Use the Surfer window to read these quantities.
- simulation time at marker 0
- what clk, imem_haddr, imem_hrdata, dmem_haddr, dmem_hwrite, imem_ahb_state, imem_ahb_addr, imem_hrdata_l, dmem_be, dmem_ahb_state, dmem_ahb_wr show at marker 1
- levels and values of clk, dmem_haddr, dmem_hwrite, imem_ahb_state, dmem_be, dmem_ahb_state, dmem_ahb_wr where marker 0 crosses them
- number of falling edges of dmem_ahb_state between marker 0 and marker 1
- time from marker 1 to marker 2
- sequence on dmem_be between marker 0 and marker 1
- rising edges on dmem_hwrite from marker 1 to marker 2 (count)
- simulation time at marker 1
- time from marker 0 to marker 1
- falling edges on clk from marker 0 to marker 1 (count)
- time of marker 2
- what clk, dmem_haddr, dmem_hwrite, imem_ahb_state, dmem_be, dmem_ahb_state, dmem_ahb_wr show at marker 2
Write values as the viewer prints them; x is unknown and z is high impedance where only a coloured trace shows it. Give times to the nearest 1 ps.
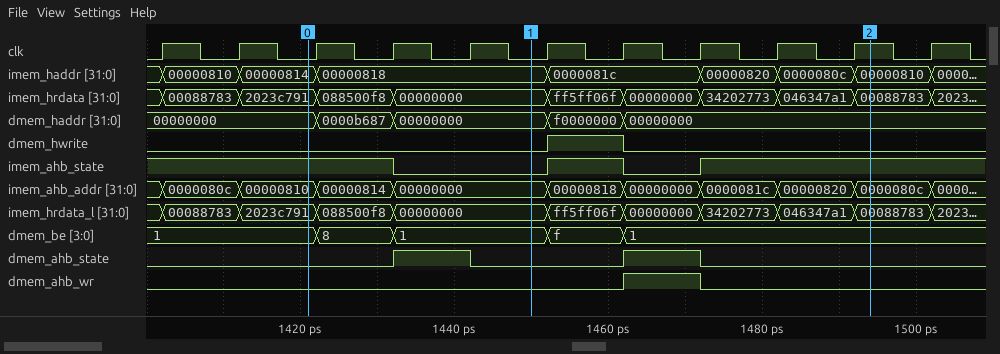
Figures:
1421 ps
clk=0, imem_haddr=00000818, imem_hrdata=00000000, dmem_haddr=00000000, dmem_hwrite=0, imem_ahb_state=0, imem_ahb_addr=00000000, imem_hrdata_l=00000000, dmem_be=1, dmem_ahb_state=0, dmem_ahb_wr=0
clk=0, dmem_haddr=00000000, dmem_hwrite=0, imem_ahb_state=1, dmem_be=1, dmem_ahb_state=0, dmem_ahb_wr=0
1
44 ps
1, 8, 1
1
1450 ps
29 ps
3
1494 ps
clk=1, dmem_haddr=00000000, dmem_hwrite=0, imem_ahb_state=1, dmem_be=1, dmem_ahb_state=0, dmem_ahb_wr=0
